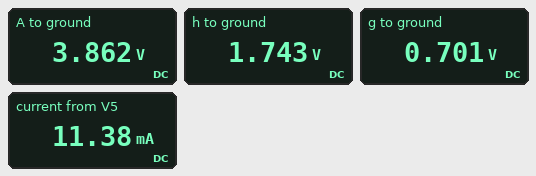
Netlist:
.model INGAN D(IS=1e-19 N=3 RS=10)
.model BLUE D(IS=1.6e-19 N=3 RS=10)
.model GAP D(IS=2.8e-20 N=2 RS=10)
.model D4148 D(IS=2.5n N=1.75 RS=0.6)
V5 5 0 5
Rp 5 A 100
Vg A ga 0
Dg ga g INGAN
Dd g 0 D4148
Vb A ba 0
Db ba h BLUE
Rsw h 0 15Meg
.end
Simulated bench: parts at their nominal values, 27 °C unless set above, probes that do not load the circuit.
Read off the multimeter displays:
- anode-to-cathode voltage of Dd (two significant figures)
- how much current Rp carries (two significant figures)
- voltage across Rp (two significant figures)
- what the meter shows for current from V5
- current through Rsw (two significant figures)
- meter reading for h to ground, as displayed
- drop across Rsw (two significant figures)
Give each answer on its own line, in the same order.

700 mV
11 mA
1.1 V
11.38 mA
120 nA
1.743 V
1.7 V
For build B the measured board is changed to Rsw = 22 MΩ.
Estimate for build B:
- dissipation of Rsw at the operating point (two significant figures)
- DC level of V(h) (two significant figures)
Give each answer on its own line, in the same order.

140 nW
1.8 V
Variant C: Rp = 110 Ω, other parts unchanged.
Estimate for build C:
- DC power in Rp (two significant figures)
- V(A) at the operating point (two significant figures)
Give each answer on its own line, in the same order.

12 mW
3.8 V
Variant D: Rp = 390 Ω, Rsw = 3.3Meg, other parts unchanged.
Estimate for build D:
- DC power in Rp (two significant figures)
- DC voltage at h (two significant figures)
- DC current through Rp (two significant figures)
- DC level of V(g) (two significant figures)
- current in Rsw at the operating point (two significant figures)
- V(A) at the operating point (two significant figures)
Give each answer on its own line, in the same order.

4.8 mW
1.4 V
3.5 mA
640 mV
430 nA
3.6 V
